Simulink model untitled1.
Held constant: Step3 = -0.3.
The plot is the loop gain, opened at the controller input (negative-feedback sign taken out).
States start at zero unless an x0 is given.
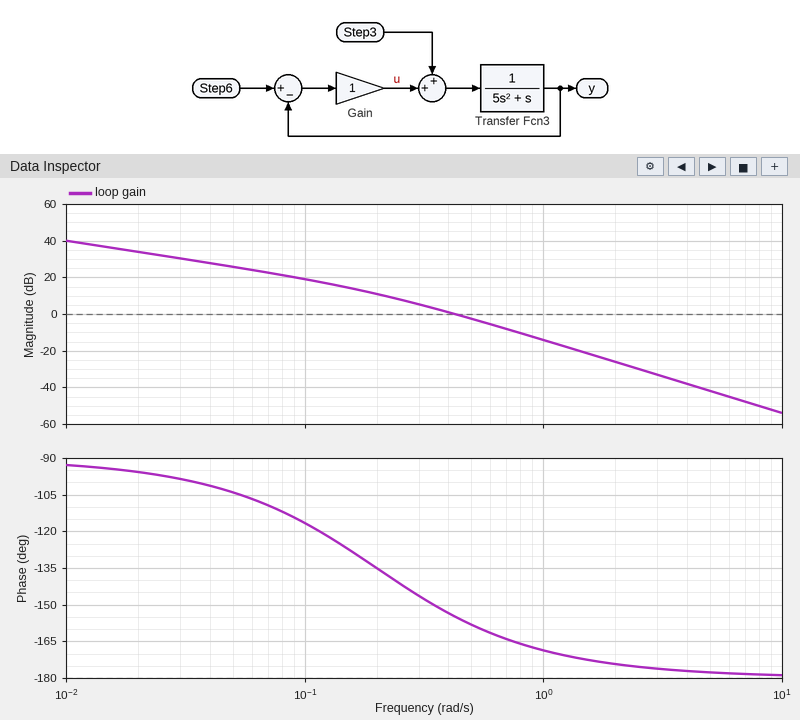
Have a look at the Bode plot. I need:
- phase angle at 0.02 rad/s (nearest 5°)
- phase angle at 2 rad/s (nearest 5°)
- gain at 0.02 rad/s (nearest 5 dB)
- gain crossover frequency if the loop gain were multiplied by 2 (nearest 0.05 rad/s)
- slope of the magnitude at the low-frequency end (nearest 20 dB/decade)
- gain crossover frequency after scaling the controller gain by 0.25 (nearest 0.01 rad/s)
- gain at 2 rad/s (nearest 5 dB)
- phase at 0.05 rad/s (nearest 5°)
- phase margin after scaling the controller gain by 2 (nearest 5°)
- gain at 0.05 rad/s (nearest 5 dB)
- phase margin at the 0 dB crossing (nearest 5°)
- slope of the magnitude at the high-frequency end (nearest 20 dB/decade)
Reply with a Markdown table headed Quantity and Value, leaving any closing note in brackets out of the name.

| Quantity | Value |
|---|---|
| phase angle at 0.02 rad/s | -95° |
| phase angle at 2 rad/s | -175° |
| gain at 0.02 rad/s | 35 dB |
| gain crossover frequency if the loop gain were multiplied by 2 | 0.60 rad/s |
| slope of the magnitude at the low-frequency end | -20 dB/decade |
| gain crossover frequency after scaling the controller gain by 0.25 | 0.18 rad/s |
| gain at 2 rad/s | -25 dB |
| phase at 0.05 rad/s | -105° |
| phase margin after scaling the controller gain by 2 | 20° |
| gain at 0.05 rad/s | 25 dB |
| phase margin at the 0 dB crossing | 25° |
| slope of the magnitude at the high-frequency end | -40 dB/decade |
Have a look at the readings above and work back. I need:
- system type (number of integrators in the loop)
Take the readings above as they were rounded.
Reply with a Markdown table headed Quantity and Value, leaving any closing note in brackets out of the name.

| Quantity | Value |
|---|---|
| system type | 1 |
